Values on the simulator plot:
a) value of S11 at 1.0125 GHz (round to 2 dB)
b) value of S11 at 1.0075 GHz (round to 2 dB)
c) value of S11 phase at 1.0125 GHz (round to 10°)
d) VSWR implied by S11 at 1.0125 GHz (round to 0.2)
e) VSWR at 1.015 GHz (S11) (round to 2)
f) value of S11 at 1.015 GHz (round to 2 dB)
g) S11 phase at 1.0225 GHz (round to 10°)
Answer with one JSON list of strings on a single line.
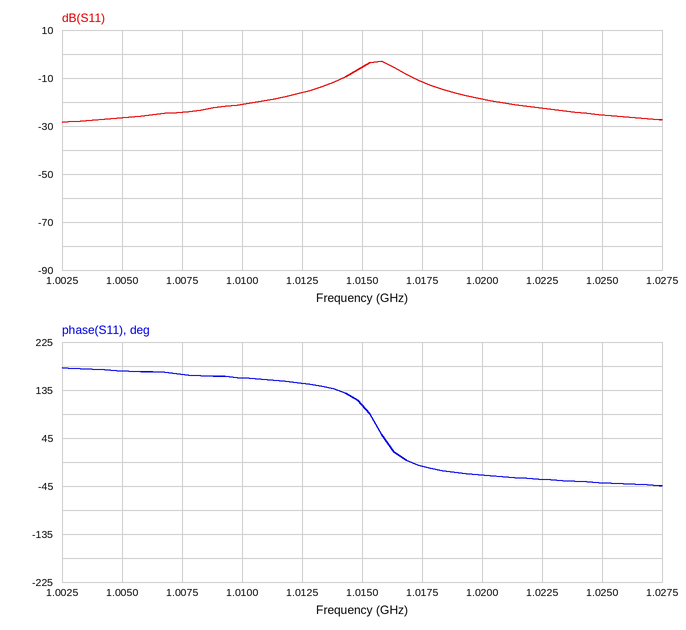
["-16 dB", "-24 dB", "150°", "1.4", "4", "-6 dB", "-30°"]
